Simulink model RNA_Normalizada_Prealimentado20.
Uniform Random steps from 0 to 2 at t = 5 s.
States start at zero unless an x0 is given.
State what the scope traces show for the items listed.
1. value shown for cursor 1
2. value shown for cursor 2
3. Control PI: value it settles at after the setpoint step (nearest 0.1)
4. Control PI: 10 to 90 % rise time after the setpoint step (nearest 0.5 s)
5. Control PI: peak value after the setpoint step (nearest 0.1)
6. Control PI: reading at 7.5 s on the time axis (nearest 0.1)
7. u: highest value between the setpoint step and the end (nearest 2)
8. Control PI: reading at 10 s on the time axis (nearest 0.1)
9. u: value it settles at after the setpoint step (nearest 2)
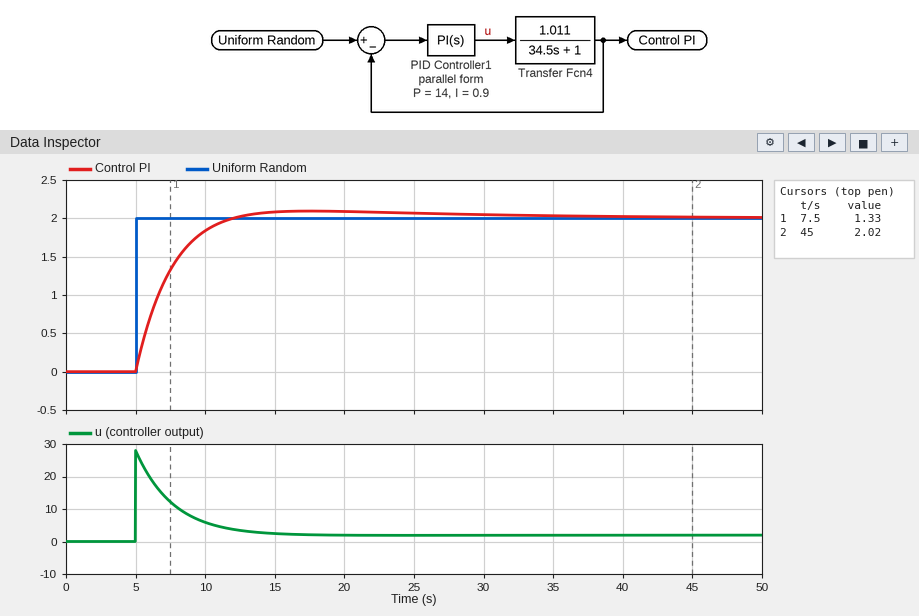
1.33
2.02
2.0
4.5 s
2.1
1.3
28
1.8
2
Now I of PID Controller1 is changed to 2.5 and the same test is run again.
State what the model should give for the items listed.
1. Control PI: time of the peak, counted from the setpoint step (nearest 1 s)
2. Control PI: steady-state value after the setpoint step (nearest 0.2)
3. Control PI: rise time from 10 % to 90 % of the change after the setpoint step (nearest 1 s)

8 s
2.0
3 s
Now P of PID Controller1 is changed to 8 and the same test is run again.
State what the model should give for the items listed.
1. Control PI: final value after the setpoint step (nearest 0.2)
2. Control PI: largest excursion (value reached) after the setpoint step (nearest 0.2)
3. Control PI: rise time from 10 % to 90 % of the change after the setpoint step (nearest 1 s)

2.0
2.2
6 s
